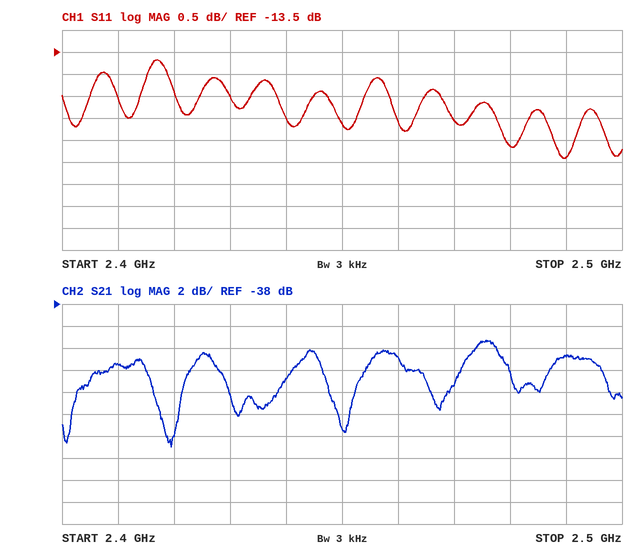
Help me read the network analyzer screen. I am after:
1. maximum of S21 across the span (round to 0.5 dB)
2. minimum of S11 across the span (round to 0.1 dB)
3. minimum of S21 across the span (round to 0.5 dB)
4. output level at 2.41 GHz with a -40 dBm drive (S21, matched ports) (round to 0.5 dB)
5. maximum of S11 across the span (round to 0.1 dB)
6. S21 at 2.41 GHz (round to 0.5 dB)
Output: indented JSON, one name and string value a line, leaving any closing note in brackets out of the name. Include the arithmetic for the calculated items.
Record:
{
  "maximum of S21 across the span": "-41.5 dB",
  "minimum of S11 across the span": "-15.9 dB",
  "minimum of S21 across the span": "-51.0 dB",
  "output level at 2.41 GHz with a -40 dBm drive (S21, matched ports)": "-40 dBm + (-43.5 dB) = -83.5 dBm",
  "maximum of S11 across the span": "-13.7 dB",
  "S21 at 2.41 GHz": "-43.5 dB"
}
